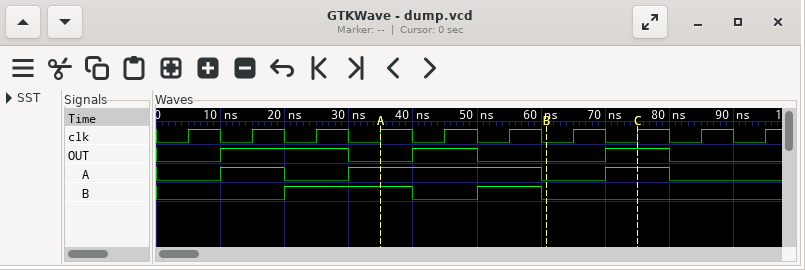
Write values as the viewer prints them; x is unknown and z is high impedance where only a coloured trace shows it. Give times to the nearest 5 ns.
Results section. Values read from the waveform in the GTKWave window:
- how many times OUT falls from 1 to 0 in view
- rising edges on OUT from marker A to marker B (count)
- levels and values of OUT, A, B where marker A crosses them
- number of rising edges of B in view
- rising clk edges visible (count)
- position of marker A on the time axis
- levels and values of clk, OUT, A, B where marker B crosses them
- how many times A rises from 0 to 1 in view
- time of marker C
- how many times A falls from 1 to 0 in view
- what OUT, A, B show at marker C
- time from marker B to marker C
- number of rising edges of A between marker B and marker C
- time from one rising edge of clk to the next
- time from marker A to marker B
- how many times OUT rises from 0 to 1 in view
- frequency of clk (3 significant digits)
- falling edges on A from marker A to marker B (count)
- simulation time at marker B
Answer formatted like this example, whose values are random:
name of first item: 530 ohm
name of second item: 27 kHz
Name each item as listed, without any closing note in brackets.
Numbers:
how many times OUT falls from 1 to 0 in view: 3
rising edges on OUT from marker A to marker B: 1
levels and values of OUT, A, B where marker A crosses them: OUT=0, A=1, B=1
number of rising edges of B in view: 2
rising clk edges visible: 10
position of marker A on the time axis: 35 ns
levels and values of clk, OUT, A, B where marker B crosses them: clk=0, OUT=0, A=0, B=0
how many times A rises from 0 to 1 in view: 3
time of marker C: 75 ns
how many times A falls from 1 to 0 in view: 3
what OUT, A, B show at marker C: OUT=1, A=1, B=0
time from marker B to marker C: 15 ns
number of rising edges of A between marker B and marker C: 1
time from one rising edge of clk to the next: 10 ns
time from marker A to marker B: 25 ns
how many times OUT rises from 0 to 1 in view: 3
frequency of clk: 100 MHz
falling edges on A from marker A to marker B: 1
simulation time at marker B: 60 ns
